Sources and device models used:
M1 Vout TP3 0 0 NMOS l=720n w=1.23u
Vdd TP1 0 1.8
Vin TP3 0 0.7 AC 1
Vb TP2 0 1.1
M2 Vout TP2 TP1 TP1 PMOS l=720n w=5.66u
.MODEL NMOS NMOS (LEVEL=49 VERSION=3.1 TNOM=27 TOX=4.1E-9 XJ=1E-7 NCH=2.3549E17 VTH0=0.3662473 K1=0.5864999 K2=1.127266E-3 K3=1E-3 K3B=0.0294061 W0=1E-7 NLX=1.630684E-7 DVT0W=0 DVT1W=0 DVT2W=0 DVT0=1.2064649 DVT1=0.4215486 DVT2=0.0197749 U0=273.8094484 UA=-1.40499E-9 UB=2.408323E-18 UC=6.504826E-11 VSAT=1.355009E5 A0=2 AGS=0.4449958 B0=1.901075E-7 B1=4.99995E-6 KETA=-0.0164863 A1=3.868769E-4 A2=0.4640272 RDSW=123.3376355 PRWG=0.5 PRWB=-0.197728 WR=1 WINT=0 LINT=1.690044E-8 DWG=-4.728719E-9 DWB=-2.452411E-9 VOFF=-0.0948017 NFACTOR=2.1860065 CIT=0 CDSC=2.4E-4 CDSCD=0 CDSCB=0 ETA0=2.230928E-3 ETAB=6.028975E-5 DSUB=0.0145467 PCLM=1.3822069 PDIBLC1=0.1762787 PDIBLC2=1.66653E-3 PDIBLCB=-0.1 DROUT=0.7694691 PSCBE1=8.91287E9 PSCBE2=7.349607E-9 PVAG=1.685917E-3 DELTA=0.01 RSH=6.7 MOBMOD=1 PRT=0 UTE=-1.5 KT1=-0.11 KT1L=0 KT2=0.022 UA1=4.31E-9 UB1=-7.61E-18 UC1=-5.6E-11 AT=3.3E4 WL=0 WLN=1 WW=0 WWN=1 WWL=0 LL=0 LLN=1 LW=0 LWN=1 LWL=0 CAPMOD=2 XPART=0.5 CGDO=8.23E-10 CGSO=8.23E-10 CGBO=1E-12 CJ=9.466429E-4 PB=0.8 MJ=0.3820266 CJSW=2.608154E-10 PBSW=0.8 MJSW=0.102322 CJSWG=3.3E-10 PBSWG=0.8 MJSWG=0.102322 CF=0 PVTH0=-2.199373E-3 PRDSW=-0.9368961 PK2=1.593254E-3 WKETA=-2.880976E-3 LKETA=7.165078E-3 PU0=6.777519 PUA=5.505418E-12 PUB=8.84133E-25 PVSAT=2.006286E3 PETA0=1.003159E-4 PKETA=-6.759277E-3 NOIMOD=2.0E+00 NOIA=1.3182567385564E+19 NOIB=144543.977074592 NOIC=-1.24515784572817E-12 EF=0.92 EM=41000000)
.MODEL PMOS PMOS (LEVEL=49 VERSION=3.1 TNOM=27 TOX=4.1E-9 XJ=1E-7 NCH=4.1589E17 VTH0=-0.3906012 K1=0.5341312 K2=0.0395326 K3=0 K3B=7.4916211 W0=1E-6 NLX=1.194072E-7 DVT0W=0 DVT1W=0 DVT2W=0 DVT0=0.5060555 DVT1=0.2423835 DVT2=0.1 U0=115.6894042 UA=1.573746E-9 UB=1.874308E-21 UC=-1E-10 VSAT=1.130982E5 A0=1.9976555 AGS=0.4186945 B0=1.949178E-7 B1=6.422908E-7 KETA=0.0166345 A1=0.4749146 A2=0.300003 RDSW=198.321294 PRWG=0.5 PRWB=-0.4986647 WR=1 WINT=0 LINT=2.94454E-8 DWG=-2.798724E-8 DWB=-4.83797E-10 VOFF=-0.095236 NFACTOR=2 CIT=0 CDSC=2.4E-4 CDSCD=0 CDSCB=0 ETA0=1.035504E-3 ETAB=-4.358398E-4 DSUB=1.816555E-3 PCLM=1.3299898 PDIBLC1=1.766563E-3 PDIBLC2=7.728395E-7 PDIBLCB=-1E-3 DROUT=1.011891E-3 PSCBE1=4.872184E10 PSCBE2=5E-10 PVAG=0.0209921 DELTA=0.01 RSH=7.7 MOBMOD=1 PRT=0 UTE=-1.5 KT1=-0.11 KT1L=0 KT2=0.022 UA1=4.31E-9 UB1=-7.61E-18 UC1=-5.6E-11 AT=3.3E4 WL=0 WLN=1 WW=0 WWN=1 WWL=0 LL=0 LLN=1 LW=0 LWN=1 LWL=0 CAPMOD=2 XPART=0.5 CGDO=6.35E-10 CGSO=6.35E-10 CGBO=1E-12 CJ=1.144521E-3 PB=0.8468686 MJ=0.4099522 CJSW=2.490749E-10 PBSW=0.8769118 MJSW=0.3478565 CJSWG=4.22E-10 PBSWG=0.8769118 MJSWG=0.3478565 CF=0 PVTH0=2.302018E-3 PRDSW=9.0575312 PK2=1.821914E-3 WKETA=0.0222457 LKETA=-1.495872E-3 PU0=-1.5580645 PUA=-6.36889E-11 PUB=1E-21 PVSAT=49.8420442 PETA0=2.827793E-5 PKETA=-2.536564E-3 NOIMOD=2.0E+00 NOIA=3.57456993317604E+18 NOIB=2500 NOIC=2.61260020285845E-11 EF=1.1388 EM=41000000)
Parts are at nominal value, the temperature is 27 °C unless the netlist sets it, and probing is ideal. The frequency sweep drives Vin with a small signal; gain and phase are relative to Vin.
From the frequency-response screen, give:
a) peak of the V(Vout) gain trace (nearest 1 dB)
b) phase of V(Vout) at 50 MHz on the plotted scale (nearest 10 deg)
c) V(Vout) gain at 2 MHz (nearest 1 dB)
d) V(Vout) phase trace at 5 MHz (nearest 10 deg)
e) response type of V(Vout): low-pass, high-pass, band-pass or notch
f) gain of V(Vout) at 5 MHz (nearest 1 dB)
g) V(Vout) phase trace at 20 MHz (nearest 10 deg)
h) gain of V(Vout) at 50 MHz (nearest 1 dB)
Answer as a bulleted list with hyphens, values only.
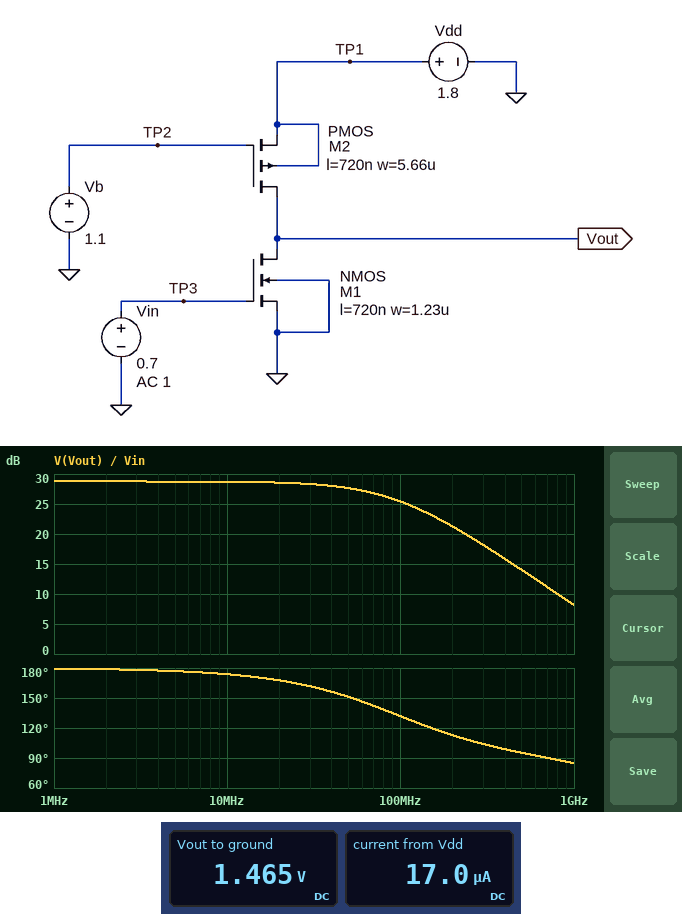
- 29 dB
- 150 deg
- 29 dB
- 180 deg
- low-pass
- 29 dB
- 170 deg
- 28 dB
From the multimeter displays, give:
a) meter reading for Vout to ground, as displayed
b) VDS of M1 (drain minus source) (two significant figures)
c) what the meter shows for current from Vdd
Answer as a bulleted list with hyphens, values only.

- 1.465 V
- 1.5 V
- 17.0 µA
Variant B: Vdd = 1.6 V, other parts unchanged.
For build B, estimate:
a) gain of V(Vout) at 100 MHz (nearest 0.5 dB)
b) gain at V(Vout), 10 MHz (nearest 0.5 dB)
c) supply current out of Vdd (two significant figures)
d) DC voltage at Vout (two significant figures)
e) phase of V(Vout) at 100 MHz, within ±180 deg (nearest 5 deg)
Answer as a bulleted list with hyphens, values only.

- -23.0 dB
- -23.5 dB
- 2.1 µA
- 16 mV
- 160 deg
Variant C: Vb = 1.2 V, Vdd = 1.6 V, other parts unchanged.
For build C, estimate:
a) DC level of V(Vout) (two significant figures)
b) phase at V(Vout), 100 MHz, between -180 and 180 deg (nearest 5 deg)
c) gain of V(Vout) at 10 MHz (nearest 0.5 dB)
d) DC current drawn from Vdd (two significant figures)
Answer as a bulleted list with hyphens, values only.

- 2.2 mV
- 110 deg
- -41.0 dB
- 290 nA
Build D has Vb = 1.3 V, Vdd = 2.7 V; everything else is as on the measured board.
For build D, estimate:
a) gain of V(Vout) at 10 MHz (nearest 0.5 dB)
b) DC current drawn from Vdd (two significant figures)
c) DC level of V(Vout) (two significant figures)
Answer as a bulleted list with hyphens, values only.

- -11.5 dB
- 18 µA
- 2.7 V
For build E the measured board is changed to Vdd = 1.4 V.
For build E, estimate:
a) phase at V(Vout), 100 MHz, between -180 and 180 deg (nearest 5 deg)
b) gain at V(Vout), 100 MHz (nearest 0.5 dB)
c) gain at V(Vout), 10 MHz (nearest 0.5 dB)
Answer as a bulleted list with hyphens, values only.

- 90 deg
- -33.5 dB
- -53.0 dB
